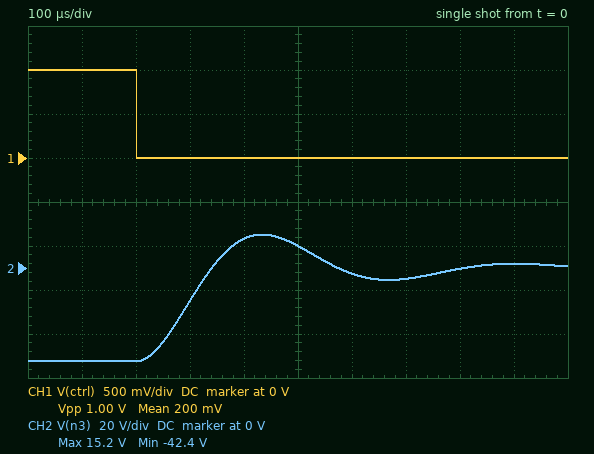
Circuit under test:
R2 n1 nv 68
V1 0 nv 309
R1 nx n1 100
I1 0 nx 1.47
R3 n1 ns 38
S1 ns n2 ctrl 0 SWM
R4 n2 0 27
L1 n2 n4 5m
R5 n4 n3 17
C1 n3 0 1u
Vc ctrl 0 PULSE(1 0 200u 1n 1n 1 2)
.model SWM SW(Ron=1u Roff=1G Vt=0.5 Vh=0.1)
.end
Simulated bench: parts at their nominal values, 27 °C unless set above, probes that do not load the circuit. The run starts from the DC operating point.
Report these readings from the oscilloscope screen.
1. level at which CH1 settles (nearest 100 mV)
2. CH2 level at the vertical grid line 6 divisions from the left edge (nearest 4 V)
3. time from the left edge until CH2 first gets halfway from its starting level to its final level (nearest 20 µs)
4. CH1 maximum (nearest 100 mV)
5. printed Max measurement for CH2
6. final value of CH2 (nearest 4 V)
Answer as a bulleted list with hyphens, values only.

- 0 V
- -4 V
- 280 µs
- 1.0 V
- 15.2 V
- 0 V
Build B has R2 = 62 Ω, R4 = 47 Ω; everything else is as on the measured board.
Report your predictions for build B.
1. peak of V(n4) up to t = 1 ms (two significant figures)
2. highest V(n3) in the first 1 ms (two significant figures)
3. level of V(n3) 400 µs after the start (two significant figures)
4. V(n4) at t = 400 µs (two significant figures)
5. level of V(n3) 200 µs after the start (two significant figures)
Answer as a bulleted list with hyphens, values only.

- 15 V
- 14 V
- 10 V
- 13 V
- -70 V
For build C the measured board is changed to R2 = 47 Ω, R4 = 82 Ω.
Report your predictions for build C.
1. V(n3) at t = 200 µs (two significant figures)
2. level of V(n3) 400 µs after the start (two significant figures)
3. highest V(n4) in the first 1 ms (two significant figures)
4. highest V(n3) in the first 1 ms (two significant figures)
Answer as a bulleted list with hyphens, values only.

- -120 V
- -7.3 V
- 5.6 V
- 5.4 V
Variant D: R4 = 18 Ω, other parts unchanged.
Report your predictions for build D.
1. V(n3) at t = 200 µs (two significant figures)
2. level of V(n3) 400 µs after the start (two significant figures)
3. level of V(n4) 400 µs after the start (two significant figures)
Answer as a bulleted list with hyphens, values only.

- -30 V
- 12 V
- 14 V
